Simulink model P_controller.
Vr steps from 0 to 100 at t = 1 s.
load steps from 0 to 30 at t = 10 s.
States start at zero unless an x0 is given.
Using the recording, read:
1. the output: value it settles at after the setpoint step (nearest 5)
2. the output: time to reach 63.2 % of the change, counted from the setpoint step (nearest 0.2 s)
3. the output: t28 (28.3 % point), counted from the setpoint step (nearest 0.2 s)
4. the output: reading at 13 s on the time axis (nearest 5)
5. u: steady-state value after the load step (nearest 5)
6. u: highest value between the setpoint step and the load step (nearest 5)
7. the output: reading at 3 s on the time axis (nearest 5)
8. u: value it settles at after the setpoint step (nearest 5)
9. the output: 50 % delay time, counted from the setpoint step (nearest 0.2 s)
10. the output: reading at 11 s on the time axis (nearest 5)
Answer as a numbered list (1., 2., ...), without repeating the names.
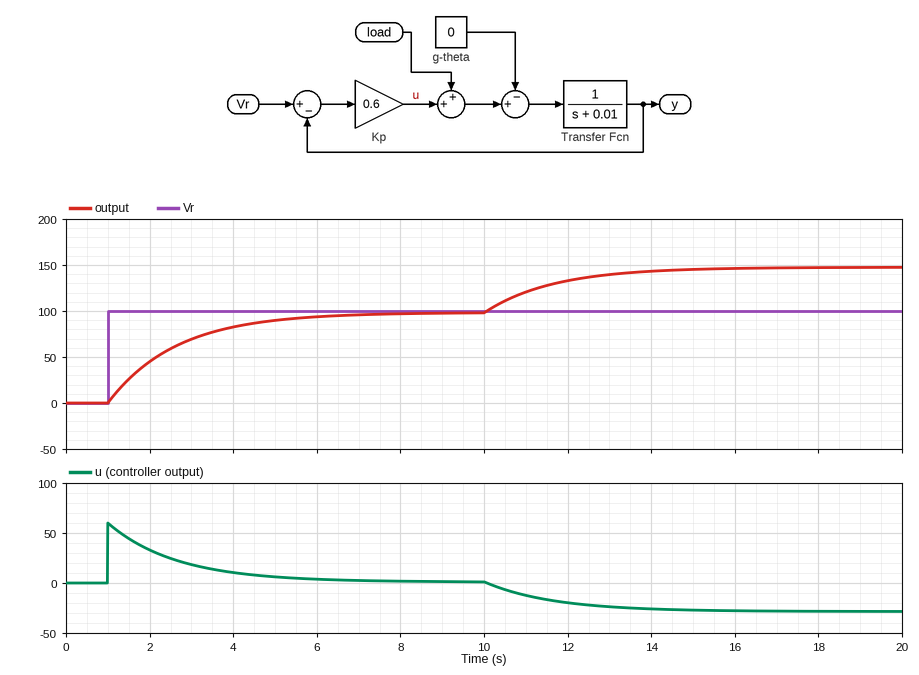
1. 100
2. 1.6 s
3. 0.6 s
4. 140
5. -30
6. 60
7. 70
8. 0
9. 1.2 s
10. 120
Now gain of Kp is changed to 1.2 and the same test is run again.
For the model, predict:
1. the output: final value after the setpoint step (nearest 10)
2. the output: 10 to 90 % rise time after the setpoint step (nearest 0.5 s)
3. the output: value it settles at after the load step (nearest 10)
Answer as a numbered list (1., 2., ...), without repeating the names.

1. 100
2. 2.0 s
3. 120
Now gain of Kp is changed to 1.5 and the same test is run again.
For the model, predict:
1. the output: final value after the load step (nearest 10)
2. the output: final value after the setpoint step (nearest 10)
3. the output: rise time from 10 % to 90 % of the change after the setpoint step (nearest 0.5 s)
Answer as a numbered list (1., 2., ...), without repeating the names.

1. 120
2. 100
3. 1.5 s
